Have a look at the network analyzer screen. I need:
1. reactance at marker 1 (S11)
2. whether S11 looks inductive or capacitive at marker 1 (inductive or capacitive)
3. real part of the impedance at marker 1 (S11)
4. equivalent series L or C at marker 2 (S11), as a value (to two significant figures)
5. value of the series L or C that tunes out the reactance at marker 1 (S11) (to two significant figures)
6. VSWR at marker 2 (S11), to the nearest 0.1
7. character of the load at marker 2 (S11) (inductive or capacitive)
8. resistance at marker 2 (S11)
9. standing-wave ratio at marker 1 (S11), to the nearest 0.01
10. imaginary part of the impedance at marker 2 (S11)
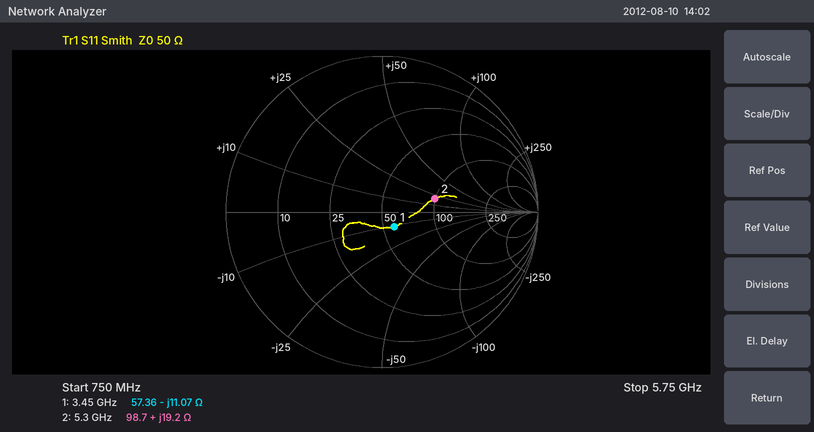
-11.07 Ω
capacitive
57.36 Ω
580 pH
510 pH
2.1
inductive
98.7 Ω
1.28
+19.2 Ω
